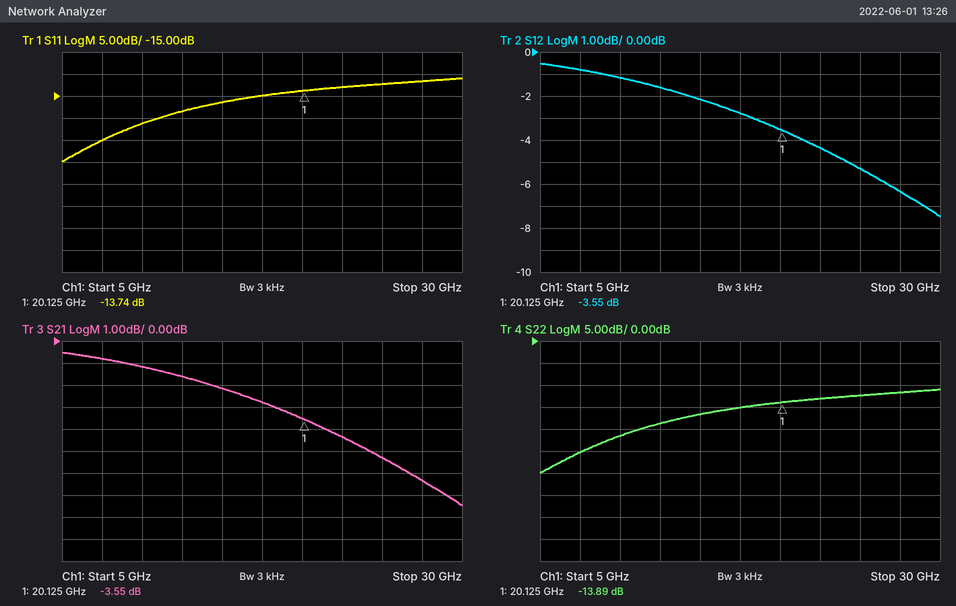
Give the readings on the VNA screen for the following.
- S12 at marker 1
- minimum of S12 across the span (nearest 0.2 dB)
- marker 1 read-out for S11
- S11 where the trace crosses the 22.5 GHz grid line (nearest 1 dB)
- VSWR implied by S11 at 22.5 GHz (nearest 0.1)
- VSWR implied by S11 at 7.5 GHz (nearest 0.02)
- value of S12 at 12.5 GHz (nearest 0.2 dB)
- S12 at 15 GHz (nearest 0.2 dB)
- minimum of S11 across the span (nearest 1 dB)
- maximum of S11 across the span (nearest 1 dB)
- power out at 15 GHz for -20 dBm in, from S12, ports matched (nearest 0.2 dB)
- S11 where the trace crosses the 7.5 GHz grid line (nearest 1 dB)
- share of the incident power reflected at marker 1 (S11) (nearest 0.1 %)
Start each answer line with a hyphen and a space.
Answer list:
- -3.55 dB
- -7.4 dB
- -13.74 dB
- -13 dB
- 1.6
- 1.12
- -1.6 dB
- -2.2 dB
- -30 dB
- -11 dB
- -22.2 dBm
- -25 dB
- 4.2 %
